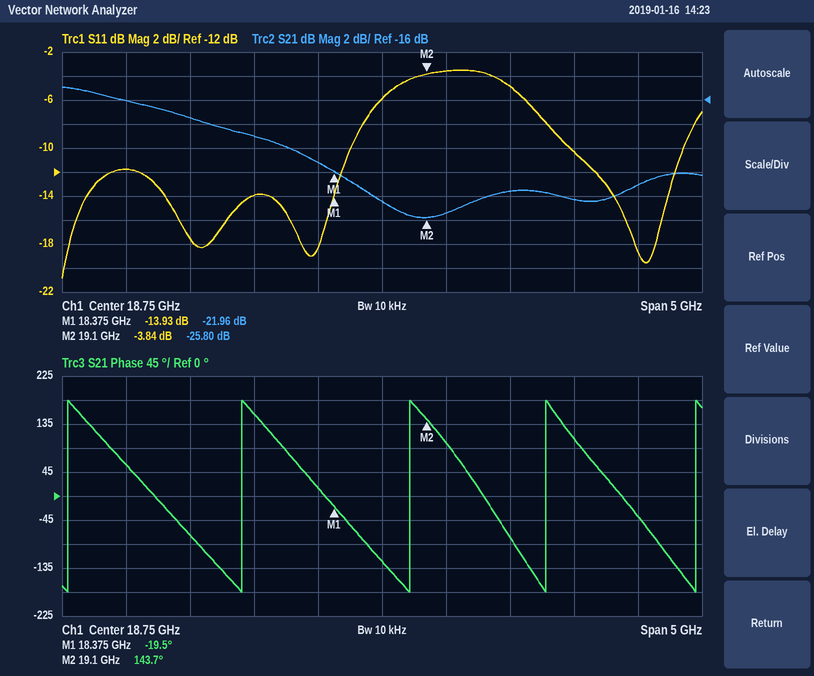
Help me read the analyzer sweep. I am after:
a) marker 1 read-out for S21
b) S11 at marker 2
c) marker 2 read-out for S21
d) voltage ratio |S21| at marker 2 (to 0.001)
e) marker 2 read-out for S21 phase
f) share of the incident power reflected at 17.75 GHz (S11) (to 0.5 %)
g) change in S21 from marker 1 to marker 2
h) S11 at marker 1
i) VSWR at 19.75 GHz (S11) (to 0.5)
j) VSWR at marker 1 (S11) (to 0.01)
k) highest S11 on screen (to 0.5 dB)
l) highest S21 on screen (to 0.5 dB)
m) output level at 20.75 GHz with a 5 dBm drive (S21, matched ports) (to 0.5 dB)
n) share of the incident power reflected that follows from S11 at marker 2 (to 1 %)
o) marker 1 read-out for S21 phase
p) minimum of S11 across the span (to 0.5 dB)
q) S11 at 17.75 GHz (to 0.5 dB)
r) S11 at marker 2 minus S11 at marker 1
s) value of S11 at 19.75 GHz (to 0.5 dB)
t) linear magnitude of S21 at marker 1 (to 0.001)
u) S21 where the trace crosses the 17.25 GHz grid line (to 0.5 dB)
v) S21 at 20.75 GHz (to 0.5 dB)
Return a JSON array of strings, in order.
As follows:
["-21.96 dB", "-3.84 dB", "-25.80 dB", "0.051", "143.7°", "4.0 %", "-3.84 dB", "-13.93 dB", "3.5", "1.50", "-3.5 dB", "-15.0 dB", "-18.0 dBm", "41 %", "-19.5°", "-21.0 dB", "-14.0 dB", "10.09 dB", "-5.0 dB", "0.080", "-17.5 dB", "-23.0 dB"]
